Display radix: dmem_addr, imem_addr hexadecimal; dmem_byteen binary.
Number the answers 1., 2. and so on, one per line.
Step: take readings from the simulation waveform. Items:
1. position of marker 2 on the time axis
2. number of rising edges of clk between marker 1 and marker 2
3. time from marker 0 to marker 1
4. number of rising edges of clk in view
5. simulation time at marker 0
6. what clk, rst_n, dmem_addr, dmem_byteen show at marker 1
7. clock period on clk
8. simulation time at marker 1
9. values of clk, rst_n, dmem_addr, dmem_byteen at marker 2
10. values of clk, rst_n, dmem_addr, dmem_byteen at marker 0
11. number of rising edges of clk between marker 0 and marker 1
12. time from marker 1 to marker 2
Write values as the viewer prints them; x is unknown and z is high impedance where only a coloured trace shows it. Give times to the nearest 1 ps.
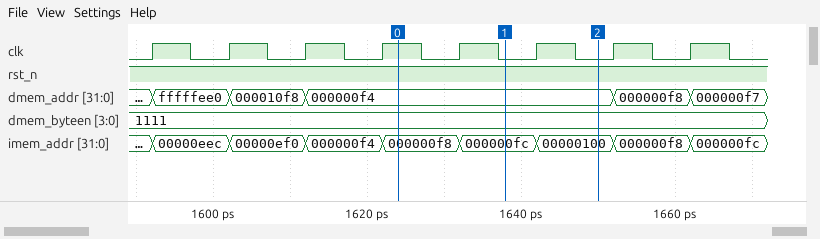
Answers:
1. 1650 ps
2. 1
3. 14 ps
4. 8
5. 1624 ps
6. clk=0, rst_n=1, dmem_addr=000000f4, dmem_byteen=1111
7. 10 ps
8. 1638 ps
9. clk=0, rst_n=1, dmem_addr=000000f4, dmem_byteen=1111
10. clk=1, rst_n=1, dmem_addr=000000f4, dmem_byteen=1111
11. 1
12. 12 ps
